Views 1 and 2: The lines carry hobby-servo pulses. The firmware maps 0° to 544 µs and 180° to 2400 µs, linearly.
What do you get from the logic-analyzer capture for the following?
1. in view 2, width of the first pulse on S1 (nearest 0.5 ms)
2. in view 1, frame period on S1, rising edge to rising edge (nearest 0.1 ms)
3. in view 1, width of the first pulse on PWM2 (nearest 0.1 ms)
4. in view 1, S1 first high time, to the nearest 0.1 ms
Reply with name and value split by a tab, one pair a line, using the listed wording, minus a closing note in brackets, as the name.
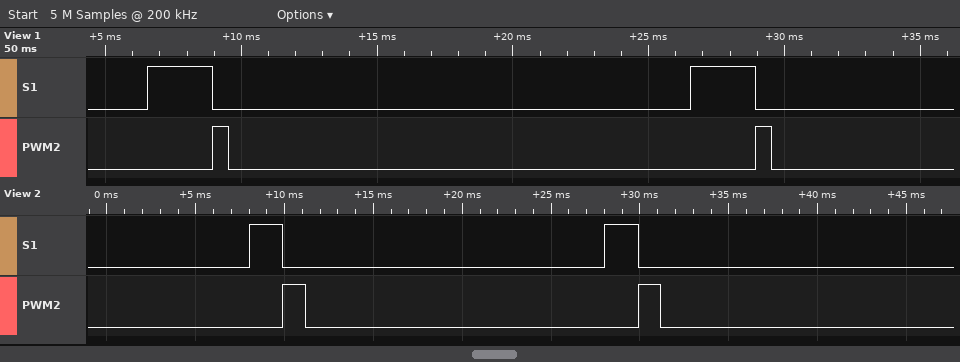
in view 2, width of the first pulse on S1	2.0 ms
in view 1, frame period on S1, rising edge to rising edge	20.0 ms
in view 1, width of the first pulse on PWM2	0.6 ms
in view 1, S1 first high time, to the nearest 0.1 ms	2.4 ms
